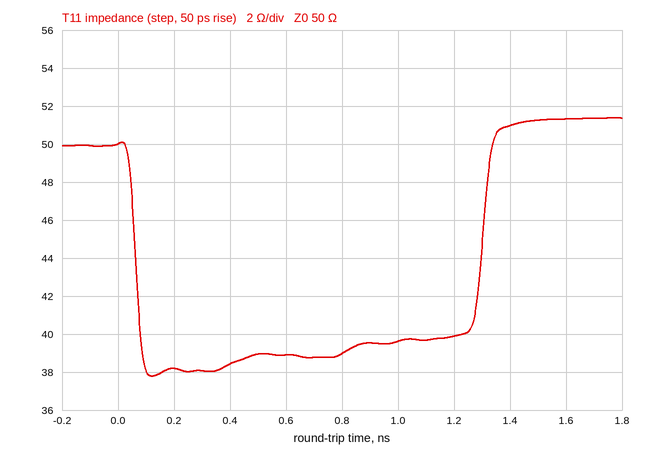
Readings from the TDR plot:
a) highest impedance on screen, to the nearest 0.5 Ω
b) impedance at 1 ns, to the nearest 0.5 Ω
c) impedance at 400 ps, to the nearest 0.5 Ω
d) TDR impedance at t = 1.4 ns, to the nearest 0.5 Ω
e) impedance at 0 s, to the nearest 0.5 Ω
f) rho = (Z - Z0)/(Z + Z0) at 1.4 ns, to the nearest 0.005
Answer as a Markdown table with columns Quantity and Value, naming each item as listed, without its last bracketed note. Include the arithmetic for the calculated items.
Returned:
| Quantity | Value |
|---|---|
| highest impedance on screen, to the nearest 0.5 Ω | 51.5 Ω |
| impedance at 1 ns, to the nearest 0.5 Ω | 39.5 Ω |
| impedance at 400 ps, to the nearest 0.5 Ω | 38.5 Ω |
| TDR impedance at t = 1.4 ns, to the nearest 0.5 Ω | 51.0 Ω |
| impedance at 0 s, to the nearest 0.5 Ω | 50.0 Ω |
| rho = (Z - Z0)/(Z + Z0) at 1.4 ns, to the nearest 0.005 | (51 − 50)/(51 + 50) ≈ +0.010 |
